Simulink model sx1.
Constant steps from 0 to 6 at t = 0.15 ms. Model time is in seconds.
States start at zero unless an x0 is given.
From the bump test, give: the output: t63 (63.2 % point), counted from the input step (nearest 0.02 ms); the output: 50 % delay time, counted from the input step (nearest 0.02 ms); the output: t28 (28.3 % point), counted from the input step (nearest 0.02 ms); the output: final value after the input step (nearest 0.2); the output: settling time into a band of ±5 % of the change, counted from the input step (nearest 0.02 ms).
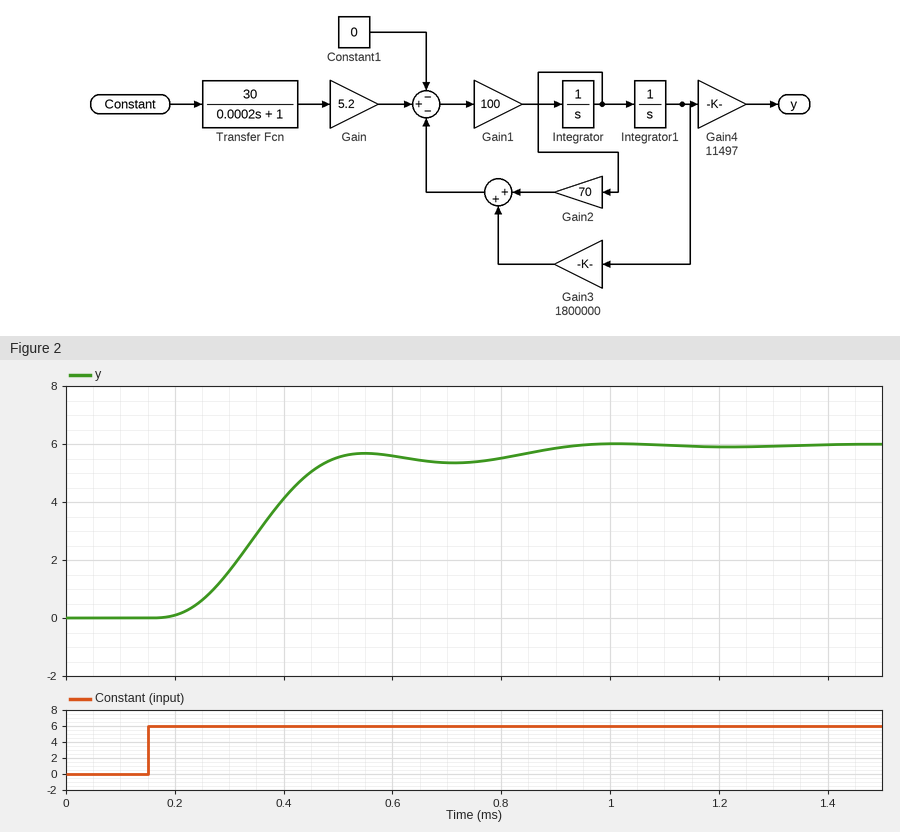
0.24 ms
0.20 ms
0.16 ms
6.0
0.70 ms
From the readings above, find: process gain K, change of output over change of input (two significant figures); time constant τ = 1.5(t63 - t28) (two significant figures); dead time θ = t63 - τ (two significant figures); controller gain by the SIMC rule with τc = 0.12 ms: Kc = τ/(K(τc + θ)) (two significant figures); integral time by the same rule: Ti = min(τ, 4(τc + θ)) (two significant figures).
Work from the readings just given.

1.0
0.12 ms
0.12 ms
0.50
0.12 ms
